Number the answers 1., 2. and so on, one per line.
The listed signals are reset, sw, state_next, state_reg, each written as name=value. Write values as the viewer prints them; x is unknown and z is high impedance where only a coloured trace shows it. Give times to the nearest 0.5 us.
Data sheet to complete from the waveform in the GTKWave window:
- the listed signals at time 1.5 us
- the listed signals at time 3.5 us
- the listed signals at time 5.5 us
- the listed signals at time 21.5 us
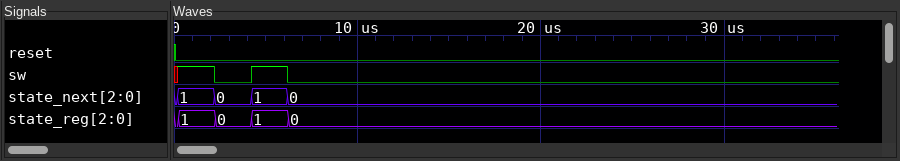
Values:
1. reset=0, sw=1, state_next=1, state_reg=1
2. reset=0, sw=0, state_next=0, state_reg=0
3. reset=0, sw=1, state_next=1, state_reg=1
4. reset=0, sw=0, state_next=0, state_reg=0
